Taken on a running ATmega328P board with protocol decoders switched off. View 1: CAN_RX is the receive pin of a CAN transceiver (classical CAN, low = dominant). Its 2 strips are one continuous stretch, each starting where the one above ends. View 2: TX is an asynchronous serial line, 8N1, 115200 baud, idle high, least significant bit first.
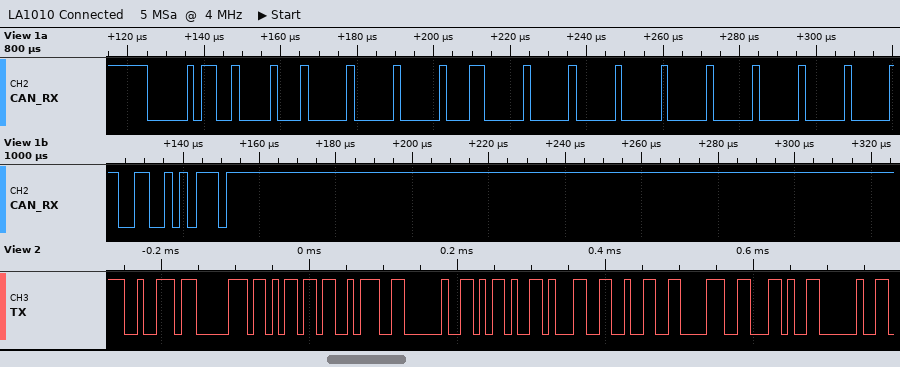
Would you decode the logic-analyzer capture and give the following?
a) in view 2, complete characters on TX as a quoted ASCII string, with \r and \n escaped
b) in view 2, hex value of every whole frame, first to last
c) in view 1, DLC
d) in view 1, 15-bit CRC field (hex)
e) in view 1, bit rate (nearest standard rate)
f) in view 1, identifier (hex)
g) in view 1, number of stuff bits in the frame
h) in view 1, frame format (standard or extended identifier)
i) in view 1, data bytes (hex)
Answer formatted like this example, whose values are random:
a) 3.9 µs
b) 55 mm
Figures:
a) "rpm: -128, "
b) 0x72 0x70 0x6D 0x3A 0x20 0x2D 0x31 0x32 0x38 0x2C 0x20
c) 8
d) 0x132B
e) 500 kbit/s
f) 0x032
g) 13
h) standard
i) 80 00 18 00 00 00 00 00
